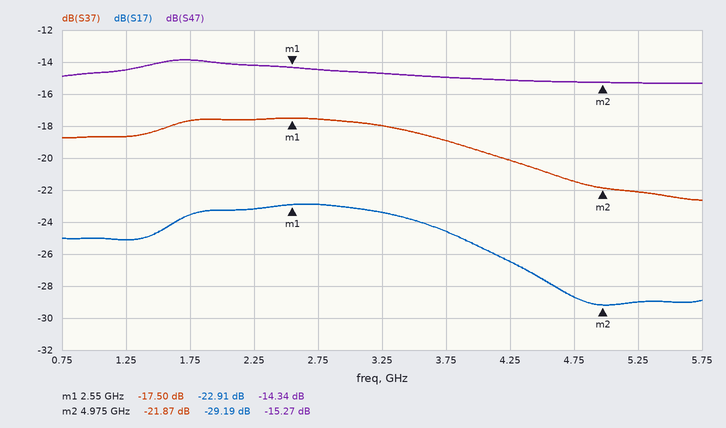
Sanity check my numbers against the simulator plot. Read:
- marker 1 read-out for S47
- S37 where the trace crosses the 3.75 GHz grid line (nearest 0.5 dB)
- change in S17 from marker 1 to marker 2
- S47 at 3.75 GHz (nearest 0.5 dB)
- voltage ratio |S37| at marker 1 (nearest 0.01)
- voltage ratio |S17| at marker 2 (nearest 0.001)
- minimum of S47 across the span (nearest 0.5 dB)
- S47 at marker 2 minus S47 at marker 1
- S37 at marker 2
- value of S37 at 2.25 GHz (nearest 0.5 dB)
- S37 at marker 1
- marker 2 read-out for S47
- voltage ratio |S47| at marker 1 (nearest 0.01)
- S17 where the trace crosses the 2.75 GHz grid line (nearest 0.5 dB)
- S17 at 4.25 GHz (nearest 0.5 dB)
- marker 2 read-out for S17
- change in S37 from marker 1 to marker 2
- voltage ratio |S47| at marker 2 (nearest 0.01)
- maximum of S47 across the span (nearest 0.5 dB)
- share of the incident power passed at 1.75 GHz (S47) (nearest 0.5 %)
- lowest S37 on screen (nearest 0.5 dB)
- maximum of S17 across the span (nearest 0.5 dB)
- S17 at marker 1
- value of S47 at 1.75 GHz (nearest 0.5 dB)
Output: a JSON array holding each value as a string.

["-14.34 dB", "-19.0 dB", "-6.28 dB", "-15.0 dB", "0.13", "0.035", "-15.5 dB", "-0.93 dB", "-21.87 dB", "-17.5 dB", "-17.50 dB", "-15.27 dB", "0.19", "-23.0 dB", "-26.5 dB", "-29.19 dB", "-4.37 dB", "0.17", "-14.0 dB", "4.0 %", "-22.5 dB", "-23.0 dB", "-22.91 dB", "-14.0 dB"]
